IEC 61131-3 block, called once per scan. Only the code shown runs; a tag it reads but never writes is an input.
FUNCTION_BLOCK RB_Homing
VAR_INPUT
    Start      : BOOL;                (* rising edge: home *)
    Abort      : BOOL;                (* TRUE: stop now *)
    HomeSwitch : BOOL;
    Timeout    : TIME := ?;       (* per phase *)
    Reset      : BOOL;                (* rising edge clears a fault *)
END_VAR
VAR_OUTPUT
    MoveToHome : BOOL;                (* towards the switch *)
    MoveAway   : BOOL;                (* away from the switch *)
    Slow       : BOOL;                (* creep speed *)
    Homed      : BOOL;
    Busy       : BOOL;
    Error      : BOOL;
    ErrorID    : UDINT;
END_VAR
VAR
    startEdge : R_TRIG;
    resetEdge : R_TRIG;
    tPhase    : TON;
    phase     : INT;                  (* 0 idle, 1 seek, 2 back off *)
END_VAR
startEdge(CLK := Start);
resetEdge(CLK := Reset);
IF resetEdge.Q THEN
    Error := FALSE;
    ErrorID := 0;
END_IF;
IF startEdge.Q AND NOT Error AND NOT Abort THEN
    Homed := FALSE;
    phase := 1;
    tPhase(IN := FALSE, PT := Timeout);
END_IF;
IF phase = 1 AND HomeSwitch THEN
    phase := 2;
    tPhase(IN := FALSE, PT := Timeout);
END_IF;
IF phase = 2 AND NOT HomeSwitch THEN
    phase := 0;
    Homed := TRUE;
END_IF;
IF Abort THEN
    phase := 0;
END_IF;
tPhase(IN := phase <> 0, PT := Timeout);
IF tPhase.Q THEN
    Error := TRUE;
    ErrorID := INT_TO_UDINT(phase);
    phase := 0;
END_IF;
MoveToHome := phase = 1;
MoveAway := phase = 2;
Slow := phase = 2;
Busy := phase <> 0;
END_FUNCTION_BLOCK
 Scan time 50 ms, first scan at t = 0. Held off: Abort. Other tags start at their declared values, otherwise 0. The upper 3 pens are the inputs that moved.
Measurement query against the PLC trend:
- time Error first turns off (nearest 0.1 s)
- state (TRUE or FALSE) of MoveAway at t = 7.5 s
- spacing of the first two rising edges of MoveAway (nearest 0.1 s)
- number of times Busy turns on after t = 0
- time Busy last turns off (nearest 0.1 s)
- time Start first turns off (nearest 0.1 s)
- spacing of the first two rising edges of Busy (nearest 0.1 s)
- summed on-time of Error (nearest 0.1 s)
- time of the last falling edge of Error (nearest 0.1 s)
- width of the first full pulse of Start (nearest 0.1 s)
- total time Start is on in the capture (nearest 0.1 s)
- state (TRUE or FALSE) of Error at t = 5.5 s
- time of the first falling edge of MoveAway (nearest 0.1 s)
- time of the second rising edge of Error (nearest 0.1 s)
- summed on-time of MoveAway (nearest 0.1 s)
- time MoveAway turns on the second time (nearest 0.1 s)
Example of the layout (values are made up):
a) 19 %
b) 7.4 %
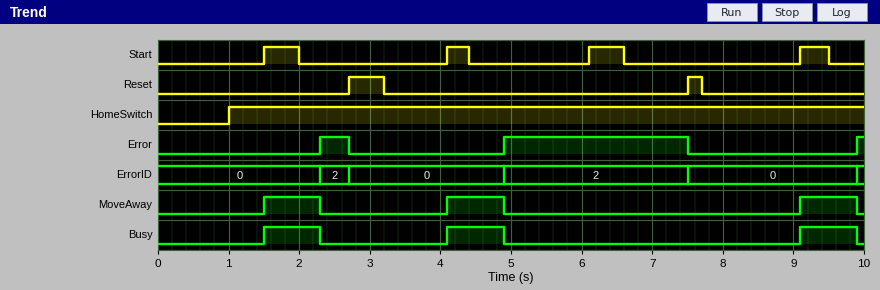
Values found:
a) 2.7 s
b) FALSE
c) 2.6 s
d) 3
e) 9.9 s
f) 2.0 s
g) 2.6 s
h) 3.1 s
i) 7.5 s
j) 0.5 s
k) 1.7 s
l) TRUE
m) 2.3 s
n) 4.9 s
o) 2.4 s
p) 4.1 s
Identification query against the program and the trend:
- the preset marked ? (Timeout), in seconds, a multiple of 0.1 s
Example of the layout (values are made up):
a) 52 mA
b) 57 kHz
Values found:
a) 0.8 s
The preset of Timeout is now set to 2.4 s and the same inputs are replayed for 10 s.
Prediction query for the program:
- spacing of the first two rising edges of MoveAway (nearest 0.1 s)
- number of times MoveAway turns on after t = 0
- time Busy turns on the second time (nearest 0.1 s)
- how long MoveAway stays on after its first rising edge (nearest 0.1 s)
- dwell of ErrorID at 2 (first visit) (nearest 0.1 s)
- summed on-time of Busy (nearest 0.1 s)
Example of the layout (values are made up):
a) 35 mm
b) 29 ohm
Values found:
a) 7.6 s
b) 2
c) 9.1 s
d) 2.4 s
e) 3.6 s
f) 3.3 s
